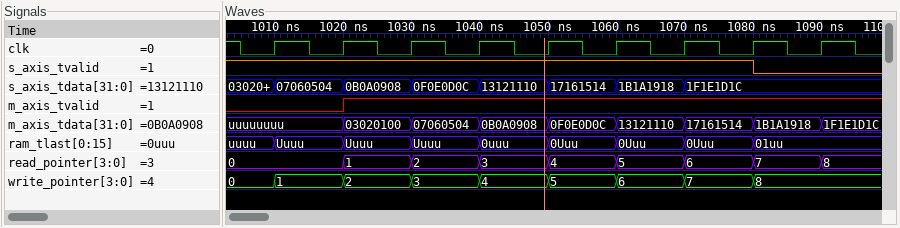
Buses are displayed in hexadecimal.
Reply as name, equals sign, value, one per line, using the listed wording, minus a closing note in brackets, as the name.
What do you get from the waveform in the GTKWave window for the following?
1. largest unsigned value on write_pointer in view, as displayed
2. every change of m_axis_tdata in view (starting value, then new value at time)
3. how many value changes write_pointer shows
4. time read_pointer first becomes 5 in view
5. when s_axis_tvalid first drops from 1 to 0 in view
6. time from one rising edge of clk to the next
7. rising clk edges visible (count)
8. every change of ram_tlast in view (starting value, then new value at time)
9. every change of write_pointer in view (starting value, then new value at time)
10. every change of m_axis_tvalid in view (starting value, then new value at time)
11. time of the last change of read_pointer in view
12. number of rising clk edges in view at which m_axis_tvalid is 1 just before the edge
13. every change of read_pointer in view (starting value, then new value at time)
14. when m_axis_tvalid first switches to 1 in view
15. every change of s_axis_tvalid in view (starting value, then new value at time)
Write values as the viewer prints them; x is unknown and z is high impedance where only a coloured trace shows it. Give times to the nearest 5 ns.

largest unsigned value on write_pointer in view, as displayed = 8
every change of m_axis_tdata in view = uuuuuuuu, 03020100 at 1020 ns, 07060504 at 1030 ns, 0B0A0908 at 1040 ns, 0F0E0D0C at 1050 ns, 13121110 at 1060 ns, 17161514 at 1070 ns, 1B1A1918 at 1080 ns, 1F1E1D1C at 1090 ns
how many value changes write_pointer shows = 8
time read_pointer first becomes 5 in view = 1060 ns
when s_axis_tvalid first drops from 1 to 0 in view = 1080 ns
time from one rising edge of clk to the next = 10 ns
rising clk edges visible = 9
every change of ram_tlast in view = uuuu, Uuuu at 1010 ns, Uuuu at 1020 ns, Uuuu at 1030 ns, 0uuu at 1040 ns, 0Uuu at 1050 ns, 0Uuu at 1060 ns, 0Uuu at 1070 ns, 01uu at 1080 ns
every change of write_pointer in view = 0, 1 at 1010 ns, 2 at 1020 ns, 3 at 1030 ns, 4 at 1040 ns, 5 at 1050 ns, 6 at 1060 ns, 7 at 1070 ns, 8 at 1080 ns
every change of m_axis_tvalid in view = 0, 1 at 1020 ns
time of the last change of read_pointer in view = 1090 ns
number of rising clk edges in view at which m_axis_tvalid is 1 just before the edge = 7
every change of read_pointer in view = 0, 1 at 1020 ns, 2 at 1030 ns, 3 at 1040 ns, 4 at 1050 ns, 5 at 1060 ns, 6 at 1070 ns, 7 at 1080 ns, 8 at 1090 ns
when m_axis_tvalid first switches to 1 in view = 1020 ns
every change of s_axis_tvalid in view = 1, 0 at 1080 ns
